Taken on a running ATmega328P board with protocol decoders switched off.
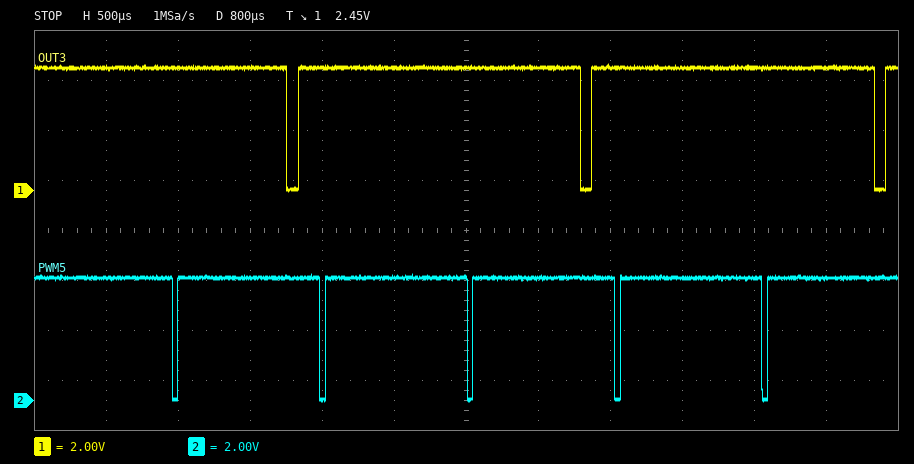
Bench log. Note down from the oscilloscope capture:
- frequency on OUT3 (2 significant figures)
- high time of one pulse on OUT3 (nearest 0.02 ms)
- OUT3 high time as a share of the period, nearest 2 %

490 Hz
1.96 ms
96 %
